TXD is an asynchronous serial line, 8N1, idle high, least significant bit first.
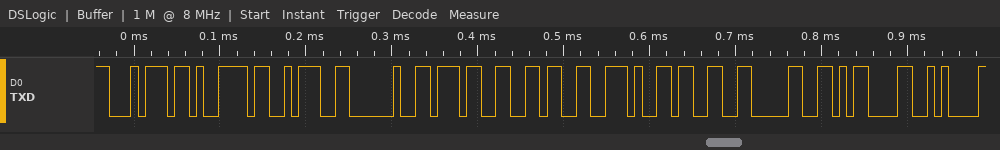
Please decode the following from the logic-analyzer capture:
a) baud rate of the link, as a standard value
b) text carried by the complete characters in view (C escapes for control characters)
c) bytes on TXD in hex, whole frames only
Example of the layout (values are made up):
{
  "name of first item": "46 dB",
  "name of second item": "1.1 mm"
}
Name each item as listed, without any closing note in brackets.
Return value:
{
  "baud rate of the link, as a standard value": "115200 baud",
  "text carried by the complete characters in view": "\"ty: 76.30\\r\\n\"",
  "bytes on TXD in hex, whole frames only": "0x74 0x79 0x3A 0x20 0x37 0x36 0x2E 0x33 0x30 0x0D 0x0A"
}
